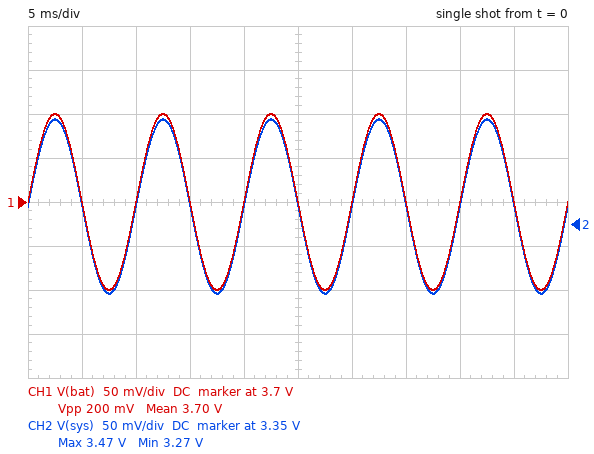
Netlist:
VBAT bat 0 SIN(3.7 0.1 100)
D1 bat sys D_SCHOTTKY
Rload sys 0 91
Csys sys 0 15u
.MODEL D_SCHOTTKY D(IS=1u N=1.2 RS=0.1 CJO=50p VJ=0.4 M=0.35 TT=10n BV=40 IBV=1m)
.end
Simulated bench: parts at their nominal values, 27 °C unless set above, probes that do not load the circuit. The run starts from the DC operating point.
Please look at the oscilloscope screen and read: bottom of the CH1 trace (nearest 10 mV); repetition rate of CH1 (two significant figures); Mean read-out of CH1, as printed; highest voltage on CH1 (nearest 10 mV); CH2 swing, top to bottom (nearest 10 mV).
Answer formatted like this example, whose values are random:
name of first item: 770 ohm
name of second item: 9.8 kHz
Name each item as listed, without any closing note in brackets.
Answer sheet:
bottom of the CH1 trace: 3.60 V
repetition rate of CH1: 100 Hz
Mean read-out of CH1, as printed: 3.70 V
highest voltage on CH1: 3.80 V
CH2 swing, top to bottom: 200 mV
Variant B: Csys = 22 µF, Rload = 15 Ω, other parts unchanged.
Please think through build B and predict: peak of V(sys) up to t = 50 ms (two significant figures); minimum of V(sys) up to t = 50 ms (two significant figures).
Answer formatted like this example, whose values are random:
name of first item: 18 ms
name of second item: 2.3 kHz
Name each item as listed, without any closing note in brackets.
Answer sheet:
peak of V(sys) up to t = 50 ms: 3.4 V
minimum of V(sys) up to t = 50 ms: 3.2 V
